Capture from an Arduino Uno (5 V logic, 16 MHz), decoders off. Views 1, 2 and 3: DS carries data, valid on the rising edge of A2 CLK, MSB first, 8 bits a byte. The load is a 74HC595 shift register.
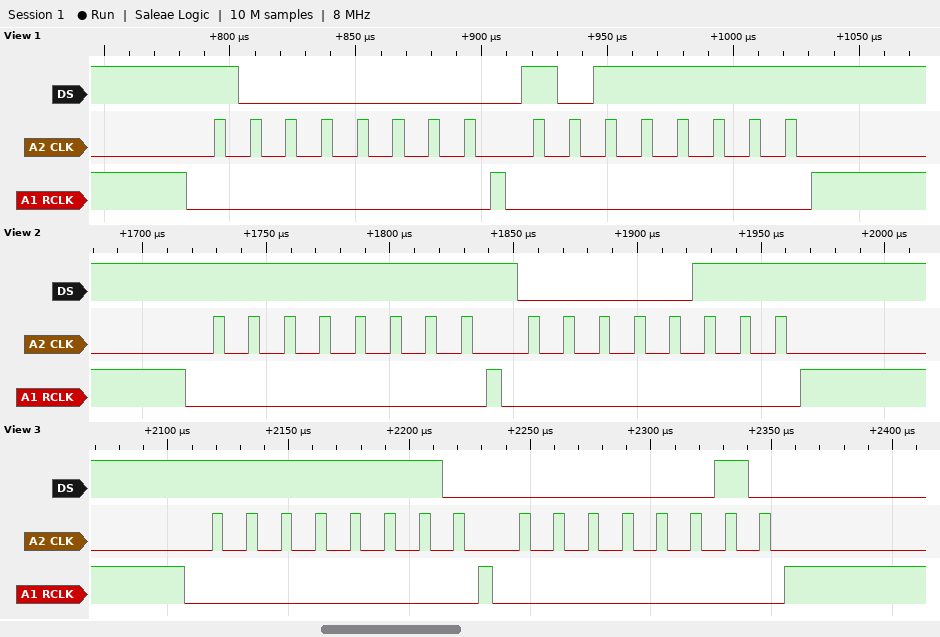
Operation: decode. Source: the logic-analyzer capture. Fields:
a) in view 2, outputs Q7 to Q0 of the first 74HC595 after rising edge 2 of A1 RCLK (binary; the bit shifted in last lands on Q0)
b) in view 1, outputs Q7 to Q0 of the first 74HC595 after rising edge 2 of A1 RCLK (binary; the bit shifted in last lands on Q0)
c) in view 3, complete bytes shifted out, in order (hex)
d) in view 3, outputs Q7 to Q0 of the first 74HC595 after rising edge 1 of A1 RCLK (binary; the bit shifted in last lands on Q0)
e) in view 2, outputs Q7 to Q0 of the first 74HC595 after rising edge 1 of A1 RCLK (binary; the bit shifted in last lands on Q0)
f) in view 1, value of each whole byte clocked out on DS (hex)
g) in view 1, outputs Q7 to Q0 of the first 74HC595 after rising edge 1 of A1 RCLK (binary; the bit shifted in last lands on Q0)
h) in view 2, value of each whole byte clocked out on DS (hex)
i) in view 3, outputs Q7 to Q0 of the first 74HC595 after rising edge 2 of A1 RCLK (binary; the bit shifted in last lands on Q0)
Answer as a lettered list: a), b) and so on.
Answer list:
a) 00000111
b) 10111111
c) FE 02
d) 11111110
e) 11111111
f) 80 BF
g) 10000000
h) FF 07
i) 00000010
